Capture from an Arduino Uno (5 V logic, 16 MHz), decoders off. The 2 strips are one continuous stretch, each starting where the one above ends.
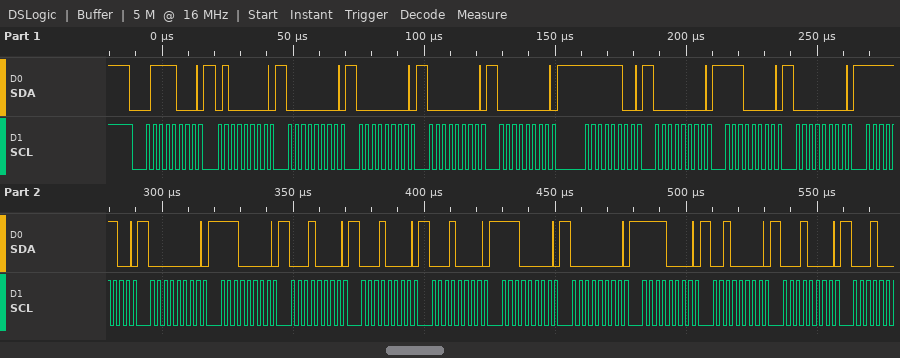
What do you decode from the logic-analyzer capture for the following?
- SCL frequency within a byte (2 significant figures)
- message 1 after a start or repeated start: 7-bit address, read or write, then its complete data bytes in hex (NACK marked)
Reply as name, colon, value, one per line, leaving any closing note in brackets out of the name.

SCL frequency within a byte: 400 kHz
message 1 after a start or repeated start: 7-bit address, read or write, then its complete data bytes in hex: 0x3C write: 40 00 00 00 00 FC 00 E0 00 FC 00 E0 10 10 10 E0 00 F0 20 10
